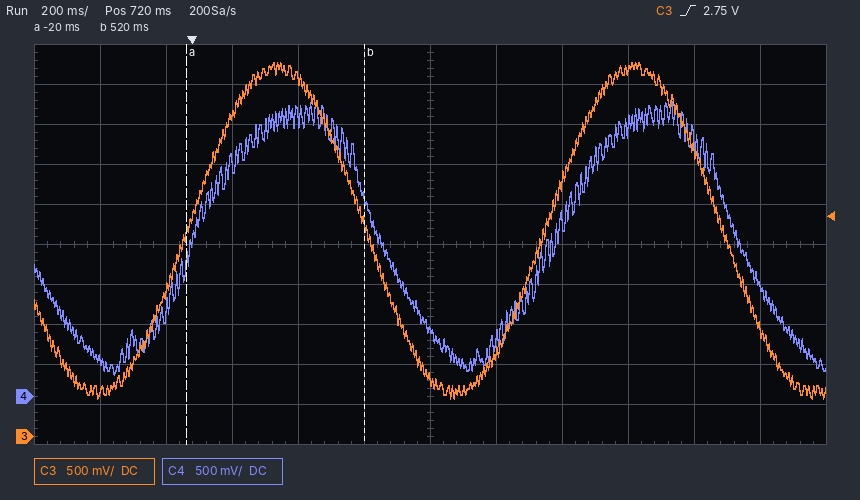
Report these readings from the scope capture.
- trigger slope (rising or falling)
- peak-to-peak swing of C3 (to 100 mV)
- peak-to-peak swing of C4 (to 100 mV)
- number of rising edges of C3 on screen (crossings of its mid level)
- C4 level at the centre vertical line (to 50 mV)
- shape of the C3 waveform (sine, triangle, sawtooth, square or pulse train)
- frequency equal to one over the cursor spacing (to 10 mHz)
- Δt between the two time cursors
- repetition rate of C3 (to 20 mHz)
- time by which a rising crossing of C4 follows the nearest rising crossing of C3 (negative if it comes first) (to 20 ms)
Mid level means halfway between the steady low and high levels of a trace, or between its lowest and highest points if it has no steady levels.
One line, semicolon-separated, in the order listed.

rising; 4.20 V; 3.40 V; 2; 850 mV; sine; 1.85 Hz; 540 ms; 920 mHz; +20 ms
